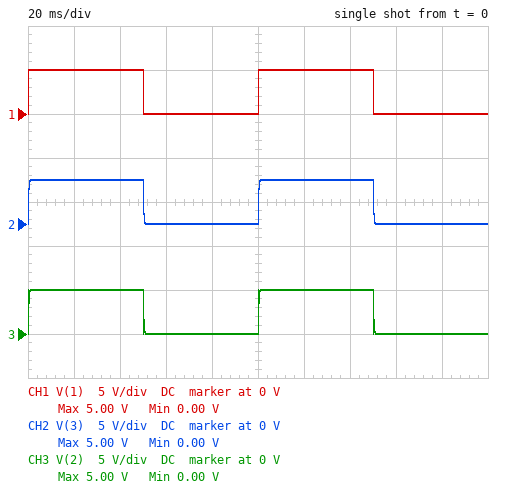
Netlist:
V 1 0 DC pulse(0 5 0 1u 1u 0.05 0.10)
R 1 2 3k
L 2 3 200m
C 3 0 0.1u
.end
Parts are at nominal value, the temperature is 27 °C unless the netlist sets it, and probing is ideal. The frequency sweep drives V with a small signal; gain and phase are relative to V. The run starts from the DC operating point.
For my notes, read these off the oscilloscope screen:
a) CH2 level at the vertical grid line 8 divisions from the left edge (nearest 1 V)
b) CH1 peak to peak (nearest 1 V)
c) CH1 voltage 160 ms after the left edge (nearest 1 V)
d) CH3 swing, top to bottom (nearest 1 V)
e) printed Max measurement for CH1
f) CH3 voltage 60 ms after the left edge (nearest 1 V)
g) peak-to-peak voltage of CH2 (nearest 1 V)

0 V
5 V
0 V
5 V
5.00 V
0 V
5 V
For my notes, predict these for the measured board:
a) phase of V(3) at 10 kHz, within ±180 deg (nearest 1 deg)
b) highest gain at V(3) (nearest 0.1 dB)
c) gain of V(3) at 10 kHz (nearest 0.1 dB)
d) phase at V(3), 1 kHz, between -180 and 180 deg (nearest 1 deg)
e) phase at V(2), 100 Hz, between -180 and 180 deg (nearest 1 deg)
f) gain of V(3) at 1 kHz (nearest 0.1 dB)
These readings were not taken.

-166 deg
0 dB
-38.1 dB
-84 deg
-11 deg
-5.6 dB
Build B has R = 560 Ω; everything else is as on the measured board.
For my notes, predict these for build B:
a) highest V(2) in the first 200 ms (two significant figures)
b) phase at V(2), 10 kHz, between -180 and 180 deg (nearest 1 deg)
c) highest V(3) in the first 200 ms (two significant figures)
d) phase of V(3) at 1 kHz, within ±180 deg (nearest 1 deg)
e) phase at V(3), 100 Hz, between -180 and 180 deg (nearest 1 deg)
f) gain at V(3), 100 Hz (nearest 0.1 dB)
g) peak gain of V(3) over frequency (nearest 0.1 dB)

5.8 V
3 deg
7.7 V
-59 deg
-2 deg
0.1 dB
8.2 dB
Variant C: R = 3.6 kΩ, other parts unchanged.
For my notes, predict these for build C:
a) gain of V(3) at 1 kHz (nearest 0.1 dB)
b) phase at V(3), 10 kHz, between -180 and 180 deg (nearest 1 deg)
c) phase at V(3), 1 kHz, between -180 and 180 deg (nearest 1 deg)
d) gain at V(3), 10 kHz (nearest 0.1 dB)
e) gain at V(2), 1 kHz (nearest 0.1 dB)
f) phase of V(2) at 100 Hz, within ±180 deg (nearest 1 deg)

-7.1 dB
-164 deg
-85 deg
-38.2 dB
-20.7 dB
-13 deg
